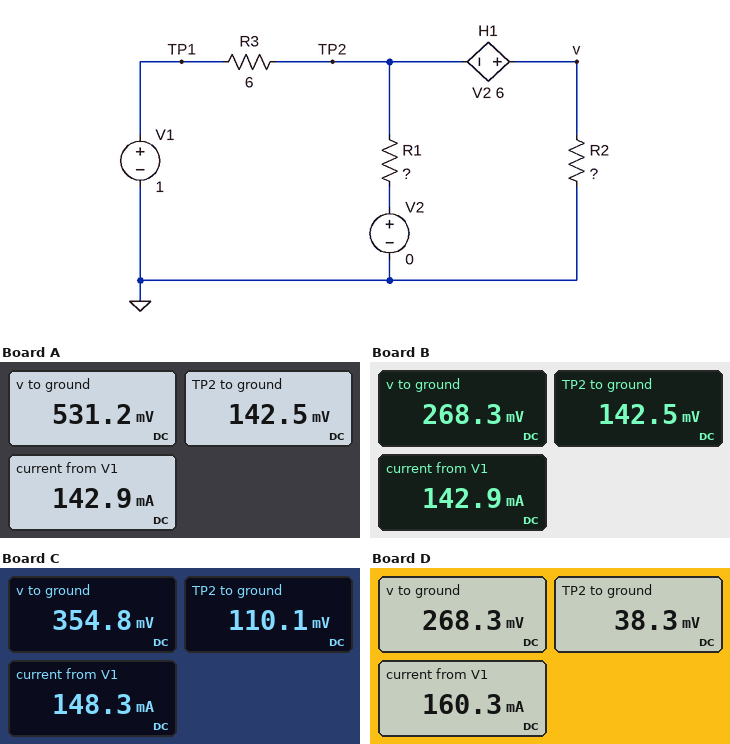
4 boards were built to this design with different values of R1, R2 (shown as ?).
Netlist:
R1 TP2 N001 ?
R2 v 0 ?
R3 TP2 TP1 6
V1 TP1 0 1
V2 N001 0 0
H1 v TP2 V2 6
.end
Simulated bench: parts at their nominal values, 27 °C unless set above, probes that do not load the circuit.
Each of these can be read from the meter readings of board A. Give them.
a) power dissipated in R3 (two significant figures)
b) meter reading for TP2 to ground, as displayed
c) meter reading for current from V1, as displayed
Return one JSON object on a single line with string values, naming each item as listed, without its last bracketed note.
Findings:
{"power dissipated in R3": "120 mW", "meter reading for TP2 to ground, as displayed": "142.5 mV", "meter reading for current from V1, as displayed": "142.9 mA"}
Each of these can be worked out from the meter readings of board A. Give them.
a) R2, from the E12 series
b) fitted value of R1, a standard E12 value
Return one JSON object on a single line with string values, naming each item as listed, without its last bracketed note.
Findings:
{"R2, from the E12 series": "6.8 Ω", "fitted value of R1, a standard E12 value": "2.2 Ω"}
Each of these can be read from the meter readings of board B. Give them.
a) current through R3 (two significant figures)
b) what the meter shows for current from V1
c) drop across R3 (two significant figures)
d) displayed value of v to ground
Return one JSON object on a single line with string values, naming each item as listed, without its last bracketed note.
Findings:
{"current through R3": "140 mA", "what the meter shows for current from V1": "142.9 mA", "drop across R3": "860 mV", "displayed value of v to ground": "268.3 mV"}
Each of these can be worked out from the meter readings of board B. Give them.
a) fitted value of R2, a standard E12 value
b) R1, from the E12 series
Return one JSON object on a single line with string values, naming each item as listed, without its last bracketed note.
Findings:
{"fitted value of R2, a standard E12 value": "2.2 Ω", "R1, from the E12 series": "6.8 Ω"}
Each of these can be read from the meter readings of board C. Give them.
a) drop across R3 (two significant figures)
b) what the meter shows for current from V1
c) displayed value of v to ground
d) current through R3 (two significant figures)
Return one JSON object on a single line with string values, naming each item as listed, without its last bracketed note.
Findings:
{"drop across R3": "890 mV", "what the meter shows for current from V1": "148.3 mA", "displayed value of v to ground": "354.8 mV", "current through R3": "150 mA"}
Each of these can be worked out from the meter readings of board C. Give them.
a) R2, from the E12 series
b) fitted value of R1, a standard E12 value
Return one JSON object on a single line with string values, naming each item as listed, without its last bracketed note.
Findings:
{"R2, from the E12 series": "3.3 Ω", "fitted value of R1, a standard E12 value": "2.7 Ω"}
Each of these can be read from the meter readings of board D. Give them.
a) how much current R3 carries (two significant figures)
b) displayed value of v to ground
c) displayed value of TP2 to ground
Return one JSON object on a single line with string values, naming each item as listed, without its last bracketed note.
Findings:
{"how much current R3 carries": "160 mA", "displayed value of v to ground": "268.3 mV", "displayed value of TP2 to ground": "38.3 mV"}
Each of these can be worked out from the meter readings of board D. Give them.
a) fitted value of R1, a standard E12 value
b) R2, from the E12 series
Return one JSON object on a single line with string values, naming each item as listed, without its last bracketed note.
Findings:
{"fitted value of R1, a standard E12 value": "1 Ω", "R2, from the E12 series": "2.2 Ω"}
